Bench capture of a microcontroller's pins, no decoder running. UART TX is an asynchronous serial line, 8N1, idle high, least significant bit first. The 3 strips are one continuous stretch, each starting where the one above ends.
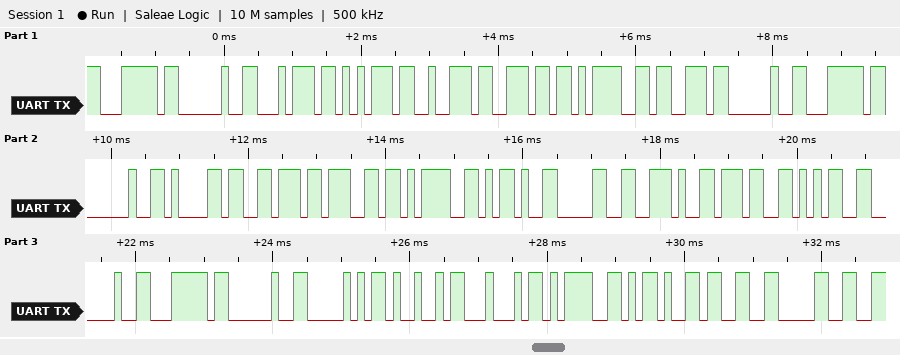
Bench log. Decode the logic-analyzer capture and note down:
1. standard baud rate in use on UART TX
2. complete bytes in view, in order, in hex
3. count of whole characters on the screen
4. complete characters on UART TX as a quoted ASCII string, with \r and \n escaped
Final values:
9600 baud
7C 20 74 75 72 6E 3D 73 20 7C 20 61 76 67 3D 2D 30 2E 37 35 20 7C 20 50 49 44 3D 2D 33 30
30
"| turn=s | avg=-0.75 | PID=-30"
